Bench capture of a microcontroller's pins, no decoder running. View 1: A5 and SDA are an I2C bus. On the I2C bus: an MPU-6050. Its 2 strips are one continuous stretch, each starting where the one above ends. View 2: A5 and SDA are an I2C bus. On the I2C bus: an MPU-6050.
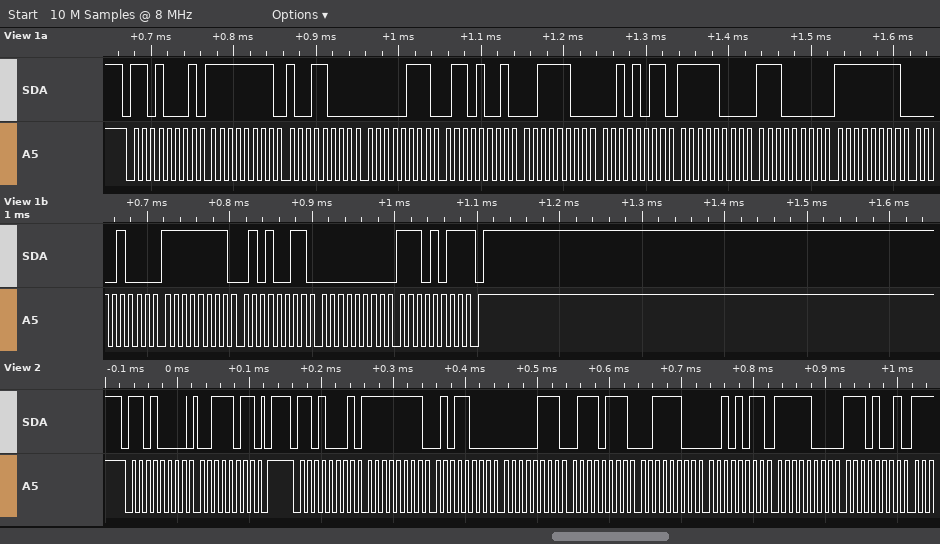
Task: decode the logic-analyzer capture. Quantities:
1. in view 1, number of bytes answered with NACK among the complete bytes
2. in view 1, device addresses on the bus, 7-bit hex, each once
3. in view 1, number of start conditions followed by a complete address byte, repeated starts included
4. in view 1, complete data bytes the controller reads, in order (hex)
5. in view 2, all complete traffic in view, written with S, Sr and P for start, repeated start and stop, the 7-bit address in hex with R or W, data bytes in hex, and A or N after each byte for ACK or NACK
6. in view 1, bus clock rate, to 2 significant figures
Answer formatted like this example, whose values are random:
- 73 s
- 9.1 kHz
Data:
- 1
- 0x68
- 1
- FF 98 07 69 3C 2B F8 E0 FF 08 FF 53 00 EB
- S 68W A 3B A P S 68R A FF A 58 A 07 A 77 A 3C A 2B A F8 A E9 A
- 100 kHz
